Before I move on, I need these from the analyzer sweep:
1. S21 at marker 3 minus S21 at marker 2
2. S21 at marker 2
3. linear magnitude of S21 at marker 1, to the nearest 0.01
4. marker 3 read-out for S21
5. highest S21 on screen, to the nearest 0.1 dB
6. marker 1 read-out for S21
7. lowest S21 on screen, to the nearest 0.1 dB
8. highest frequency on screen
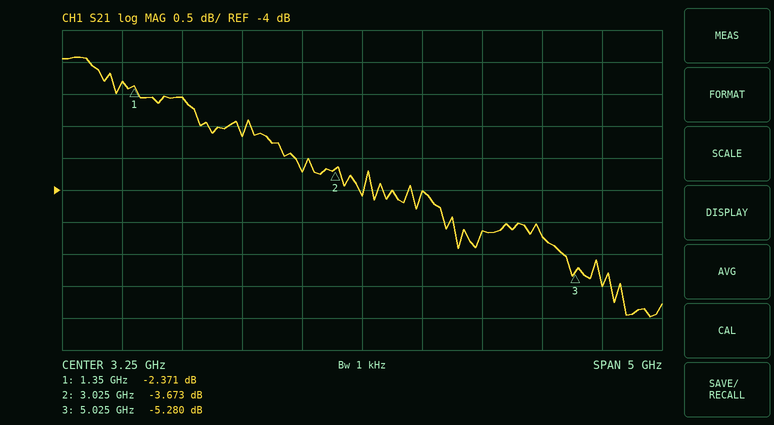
-1.607 dB
-3.673 dB
0.76
-5.280 dB
-1.9 dB
-2.371 dB
-6.0 dB
5.75 GHz
